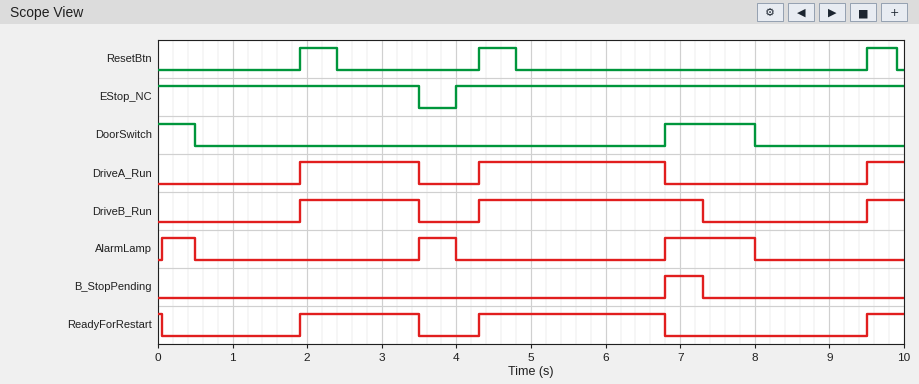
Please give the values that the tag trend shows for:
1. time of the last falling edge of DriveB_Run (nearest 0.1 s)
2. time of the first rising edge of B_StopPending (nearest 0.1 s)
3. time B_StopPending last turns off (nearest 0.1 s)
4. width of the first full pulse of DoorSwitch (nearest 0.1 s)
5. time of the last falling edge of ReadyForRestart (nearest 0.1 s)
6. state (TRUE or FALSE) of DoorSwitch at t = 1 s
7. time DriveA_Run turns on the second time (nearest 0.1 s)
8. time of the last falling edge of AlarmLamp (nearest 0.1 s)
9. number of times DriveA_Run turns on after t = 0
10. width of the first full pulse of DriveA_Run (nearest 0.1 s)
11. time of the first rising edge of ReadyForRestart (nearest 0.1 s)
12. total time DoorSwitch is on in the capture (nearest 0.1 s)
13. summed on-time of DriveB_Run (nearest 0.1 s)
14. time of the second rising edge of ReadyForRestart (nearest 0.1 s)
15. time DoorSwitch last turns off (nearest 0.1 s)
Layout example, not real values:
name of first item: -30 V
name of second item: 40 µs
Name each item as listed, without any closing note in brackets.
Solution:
time of the last falling edge of DriveB_Run: 7.3 s
time of the first rising edge of B_StopPending: 6.8 s
time B_StopPending last turns off: 7.3 s
width of the first full pulse of DoorSwitch: 1.2 s
time of the last falling edge of ReadyForRestart: 6.8 s
state (TRUE or FALSE) of DoorSwitch at t = 1 s: FALSE
time DriveA_Run turns on the second time: 4.3 s
time of the last falling edge of AlarmLamp: 8.0 s
number of times DriveA_Run turns on after t = 0: 3
width of the first full pulse of DriveA_Run: 1.6 s
time of the first rising edge of ReadyForRestart: 1.9 s
total time DoorSwitch is on in the capture: 1.7 s
summed on-time of DriveB_Run: 5.1 s
time of the second rising edge of ReadyForRestart: 4.3 s
time DoorSwitch last turns off: 8.0 s
